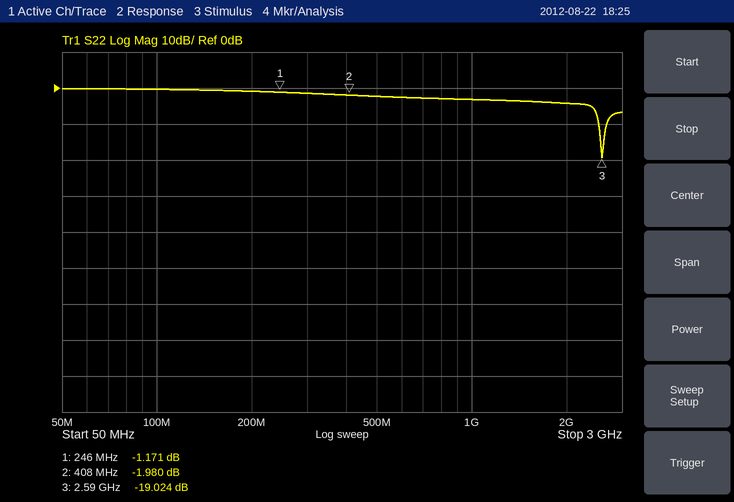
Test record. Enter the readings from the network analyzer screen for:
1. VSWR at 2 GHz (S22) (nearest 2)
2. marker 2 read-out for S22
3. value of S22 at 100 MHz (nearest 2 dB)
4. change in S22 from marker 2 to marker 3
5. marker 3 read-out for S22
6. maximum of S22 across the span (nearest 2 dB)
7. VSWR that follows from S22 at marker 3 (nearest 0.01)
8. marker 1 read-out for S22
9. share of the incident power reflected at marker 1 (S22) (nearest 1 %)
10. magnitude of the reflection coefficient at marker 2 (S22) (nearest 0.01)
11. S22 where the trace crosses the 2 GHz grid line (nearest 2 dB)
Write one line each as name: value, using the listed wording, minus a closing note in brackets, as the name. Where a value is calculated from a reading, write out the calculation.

VSWR at 2 GHz (S22): |Γ| = 10^(-4/20) = 0.6310; VSWR = (1 + 0.6310)/(1 − 0.6310) ≈ 4
marker 2 read-out for S22: -1.980 dB
value of S22 at 100 MHz: 0 dB
change in S22 from marker 2 to marker 3: -19.024 − (-1.98) = -17.044 dB
marker 3 read-out for S22: -19.024 dB
maximum of S22 across the span: 0 dB
VSWR that follows from S22 at marker 3: (1 + 0.1119)/(1 − 0.1119) ≈ 1.25
marker 1 read-out for S22: -1.171 dB
share of the incident power reflected at marker 1 (S22): 10^(-1.171/10) ≈ 76 %
magnitude of the reflection coefficient at marker 2 (S22): 10^(-1.98/20) ≈ 0.80
S22 where the trace crosses the 2 GHz grid line: -4 dB
